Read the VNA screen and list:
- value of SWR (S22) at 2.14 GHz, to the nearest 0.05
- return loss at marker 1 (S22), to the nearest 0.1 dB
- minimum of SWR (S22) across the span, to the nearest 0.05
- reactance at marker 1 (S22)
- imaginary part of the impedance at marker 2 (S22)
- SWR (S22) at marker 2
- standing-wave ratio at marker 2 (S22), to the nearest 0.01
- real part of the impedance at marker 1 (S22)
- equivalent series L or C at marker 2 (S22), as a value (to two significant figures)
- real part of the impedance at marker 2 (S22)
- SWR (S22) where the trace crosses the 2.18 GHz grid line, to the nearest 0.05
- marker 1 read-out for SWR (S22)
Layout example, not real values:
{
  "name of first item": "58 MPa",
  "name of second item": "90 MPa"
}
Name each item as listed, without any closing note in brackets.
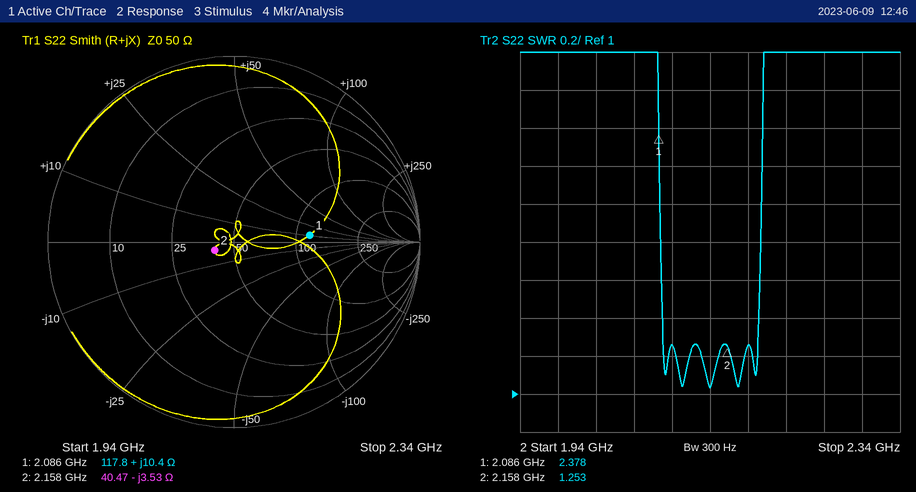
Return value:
{
  "value of SWR (S22) at 2.14 GHz, to the nearest 0.05": "1.05",
  "return loss at marker 1 (S22), to the nearest 0.1 dB": "7.8 dB",
  "minimum of SWR (S22) across the span, to the nearest 0.05": "1.05",
  "reactance at marker 1": "+10.4 Ω",
  "imaginary part of the impedance at marker 2": "-3.53 Ω",
  "SWR (S22) at marker 2": "1.253",
  "standing-wave ratio at marker 2 (S22), to the nearest 0.01": "1.25",
  "real part of the impedance at marker 1": "117.8 Ω",
  "equivalent series L or C at marker 2 (S22), as a value": "21 pF",
  "real part of the impedance at marker 2": "40.47 Ω",
  "SWR (S22) where the trace crosses the 2.18 GHz grid line, to the nearest 0.05": "1.25",
  "marker 1 read-out for SWR": "2.378"
}
